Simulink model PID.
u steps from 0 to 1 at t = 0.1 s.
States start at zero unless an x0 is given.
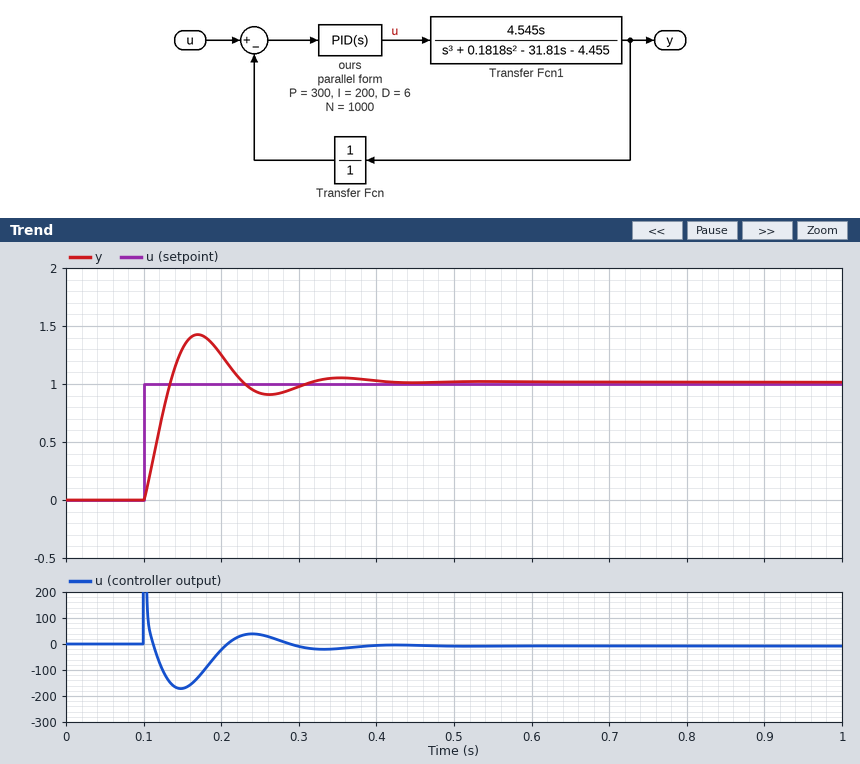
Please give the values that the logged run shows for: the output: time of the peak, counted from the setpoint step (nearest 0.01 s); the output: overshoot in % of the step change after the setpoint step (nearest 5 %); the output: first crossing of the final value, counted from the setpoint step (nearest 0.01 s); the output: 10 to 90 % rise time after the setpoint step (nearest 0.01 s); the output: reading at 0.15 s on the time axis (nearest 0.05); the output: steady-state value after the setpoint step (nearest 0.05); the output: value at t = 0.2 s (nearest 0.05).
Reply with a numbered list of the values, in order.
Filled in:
1. 0.07 s
2. 40 %
3. 0.03 s
4. 0.03 s
5. 1.30
6. 1.00
7. 1.25
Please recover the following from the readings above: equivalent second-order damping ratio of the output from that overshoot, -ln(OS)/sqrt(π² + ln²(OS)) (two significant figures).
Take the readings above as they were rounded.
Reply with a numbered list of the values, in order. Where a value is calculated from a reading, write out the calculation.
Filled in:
1. ln(0.4) = -0.916; 0.916 / sqrt(9.870 + 0.840) = 0.28
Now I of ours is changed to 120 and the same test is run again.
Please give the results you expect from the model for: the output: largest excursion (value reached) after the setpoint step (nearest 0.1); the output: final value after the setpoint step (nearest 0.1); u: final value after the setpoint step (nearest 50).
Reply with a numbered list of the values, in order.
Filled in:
1. 1.4
2. 1.0
3. 0
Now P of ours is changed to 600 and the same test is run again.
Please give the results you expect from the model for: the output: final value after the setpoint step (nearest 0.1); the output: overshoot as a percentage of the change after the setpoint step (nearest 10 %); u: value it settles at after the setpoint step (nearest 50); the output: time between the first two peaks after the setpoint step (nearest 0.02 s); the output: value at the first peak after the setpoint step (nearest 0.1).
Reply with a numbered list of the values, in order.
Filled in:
1. 1.0
2. 50 %
3. 0
4. 0.12 s
5. 1.5
